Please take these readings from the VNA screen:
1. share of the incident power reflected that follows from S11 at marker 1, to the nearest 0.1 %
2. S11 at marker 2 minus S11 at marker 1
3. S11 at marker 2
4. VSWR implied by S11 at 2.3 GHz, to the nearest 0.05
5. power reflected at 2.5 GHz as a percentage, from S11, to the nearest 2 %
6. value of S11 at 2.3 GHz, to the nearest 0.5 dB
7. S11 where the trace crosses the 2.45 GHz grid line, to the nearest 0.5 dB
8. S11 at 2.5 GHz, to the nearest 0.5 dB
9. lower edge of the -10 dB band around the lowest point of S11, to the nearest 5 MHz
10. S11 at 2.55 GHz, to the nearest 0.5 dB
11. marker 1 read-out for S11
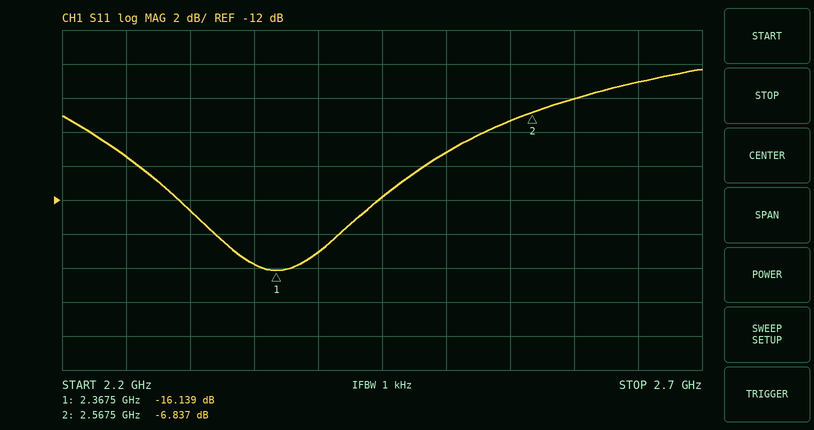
2.4 %
9.302 dB
-6.837 dB
1.60
12 %
-12.5 dB
-12.0 dB
-9.0 dB
2.260 GHz
-7.5 dB
-16.139 dB
